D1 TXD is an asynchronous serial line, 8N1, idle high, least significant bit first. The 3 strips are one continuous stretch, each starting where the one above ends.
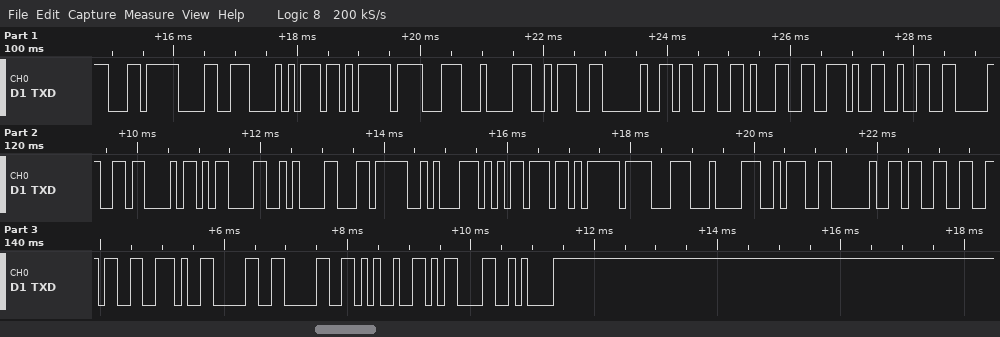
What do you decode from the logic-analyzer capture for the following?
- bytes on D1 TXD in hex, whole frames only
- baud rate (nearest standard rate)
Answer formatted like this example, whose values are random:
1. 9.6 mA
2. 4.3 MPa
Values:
1. EC 98 A8 EB 8F 84 3A 20 33 31 2E 32 30 43 0D 0A EC 8A B5 EB 8F 84 3A 20 33 36 2E 30 30 25 0D 0A
2. 9600 baud
